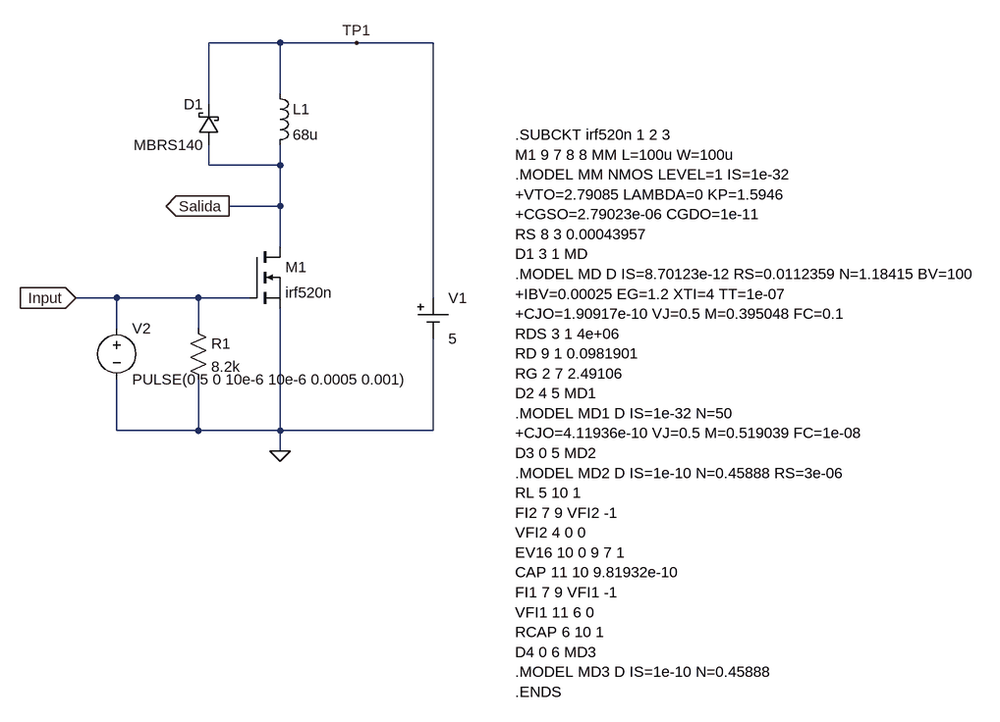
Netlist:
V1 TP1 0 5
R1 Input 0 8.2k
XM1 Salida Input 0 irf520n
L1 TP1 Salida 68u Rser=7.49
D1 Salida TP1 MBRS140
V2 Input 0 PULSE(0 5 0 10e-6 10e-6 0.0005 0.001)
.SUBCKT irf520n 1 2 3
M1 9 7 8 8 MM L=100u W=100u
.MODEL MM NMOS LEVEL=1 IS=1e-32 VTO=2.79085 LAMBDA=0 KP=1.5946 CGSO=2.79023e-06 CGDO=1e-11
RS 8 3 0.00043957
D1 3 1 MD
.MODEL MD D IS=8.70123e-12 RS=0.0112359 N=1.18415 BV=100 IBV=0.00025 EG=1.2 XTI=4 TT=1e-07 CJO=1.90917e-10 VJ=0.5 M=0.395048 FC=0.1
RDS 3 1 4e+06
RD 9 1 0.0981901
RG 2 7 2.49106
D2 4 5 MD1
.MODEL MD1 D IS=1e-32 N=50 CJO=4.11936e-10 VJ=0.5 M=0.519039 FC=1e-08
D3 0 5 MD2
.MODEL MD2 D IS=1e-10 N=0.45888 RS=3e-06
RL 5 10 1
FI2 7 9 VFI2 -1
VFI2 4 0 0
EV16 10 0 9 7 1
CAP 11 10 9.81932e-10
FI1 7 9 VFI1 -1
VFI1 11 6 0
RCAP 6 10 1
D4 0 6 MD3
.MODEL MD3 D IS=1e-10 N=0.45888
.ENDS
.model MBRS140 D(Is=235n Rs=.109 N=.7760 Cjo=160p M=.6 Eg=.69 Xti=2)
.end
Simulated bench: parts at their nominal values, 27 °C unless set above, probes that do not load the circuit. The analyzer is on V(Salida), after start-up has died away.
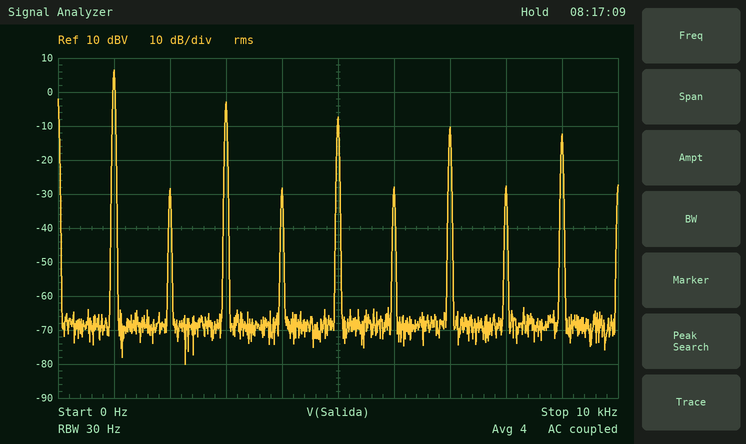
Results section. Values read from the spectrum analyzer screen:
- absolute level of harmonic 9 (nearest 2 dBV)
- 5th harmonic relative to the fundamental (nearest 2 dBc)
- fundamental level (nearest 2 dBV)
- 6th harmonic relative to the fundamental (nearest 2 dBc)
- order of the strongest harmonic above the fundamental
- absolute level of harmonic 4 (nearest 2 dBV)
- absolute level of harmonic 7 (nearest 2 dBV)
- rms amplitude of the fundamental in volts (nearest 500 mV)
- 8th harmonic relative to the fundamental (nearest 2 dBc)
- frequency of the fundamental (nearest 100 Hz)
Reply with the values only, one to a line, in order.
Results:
-12 dBV
-14 dBc
6 dBV
-34 dBc
3
-28 dBV
-10 dBV
2.0 V
-34 dBc
1.0 kHz
